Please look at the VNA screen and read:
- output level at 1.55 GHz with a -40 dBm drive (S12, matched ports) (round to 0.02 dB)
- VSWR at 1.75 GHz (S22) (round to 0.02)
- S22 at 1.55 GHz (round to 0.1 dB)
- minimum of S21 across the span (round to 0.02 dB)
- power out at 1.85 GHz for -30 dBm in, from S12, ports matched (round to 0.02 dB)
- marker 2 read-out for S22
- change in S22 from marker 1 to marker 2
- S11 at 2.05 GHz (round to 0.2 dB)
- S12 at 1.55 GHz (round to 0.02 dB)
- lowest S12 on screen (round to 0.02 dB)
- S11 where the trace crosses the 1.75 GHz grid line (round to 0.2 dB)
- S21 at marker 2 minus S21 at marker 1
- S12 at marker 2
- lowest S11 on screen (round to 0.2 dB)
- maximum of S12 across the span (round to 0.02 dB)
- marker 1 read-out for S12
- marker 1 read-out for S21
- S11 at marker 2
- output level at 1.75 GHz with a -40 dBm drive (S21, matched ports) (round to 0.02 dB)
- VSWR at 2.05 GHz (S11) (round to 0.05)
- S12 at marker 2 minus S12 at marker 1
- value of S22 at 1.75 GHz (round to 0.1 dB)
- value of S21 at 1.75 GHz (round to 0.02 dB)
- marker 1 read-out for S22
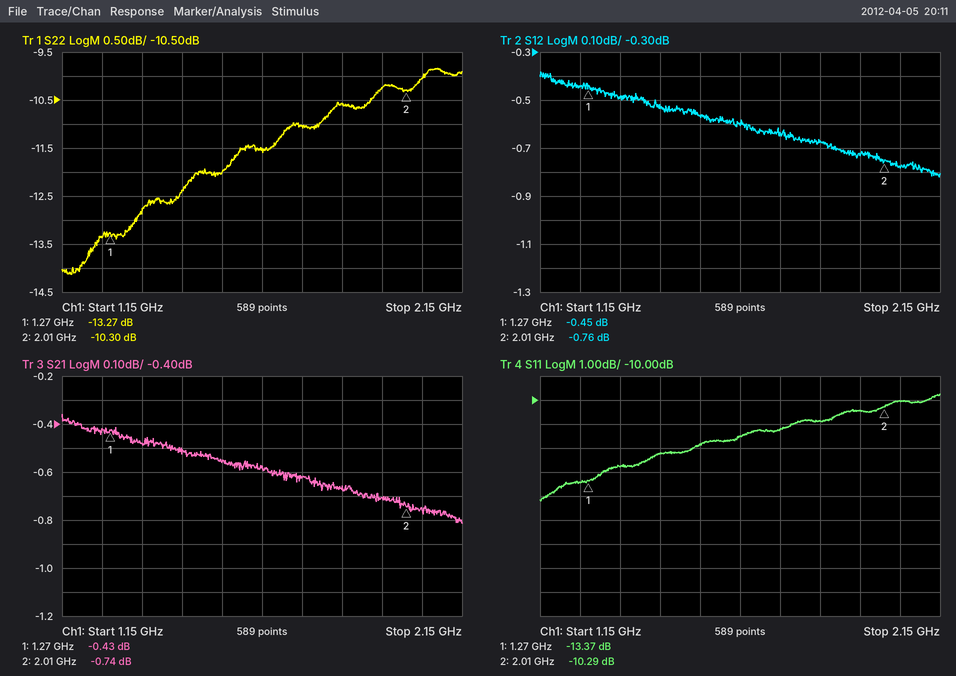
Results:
-40.56 dBm
1.78
-12.0 dB
-0.82 dB
-30.68 dBm
-10.30 dB
2.97 dB
-10.0 dB
-0.56 dB
-0.82 dB
-11.2 dB
-0.31 dB
-0.76 dB
-14.2 dB
-0.38 dB
-0.45 dB
-0.43 dB
-10.29 dB
-40.62 dBm
1.90
-0.31 dB
-11.0 dB
-0.62 dB
-13.27 dB
